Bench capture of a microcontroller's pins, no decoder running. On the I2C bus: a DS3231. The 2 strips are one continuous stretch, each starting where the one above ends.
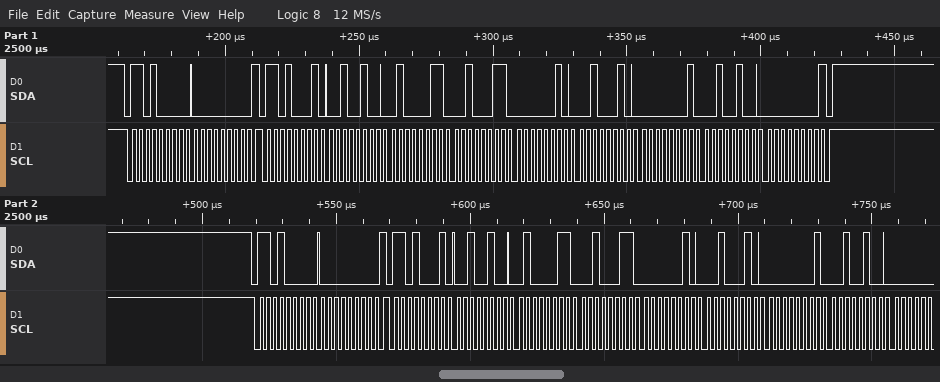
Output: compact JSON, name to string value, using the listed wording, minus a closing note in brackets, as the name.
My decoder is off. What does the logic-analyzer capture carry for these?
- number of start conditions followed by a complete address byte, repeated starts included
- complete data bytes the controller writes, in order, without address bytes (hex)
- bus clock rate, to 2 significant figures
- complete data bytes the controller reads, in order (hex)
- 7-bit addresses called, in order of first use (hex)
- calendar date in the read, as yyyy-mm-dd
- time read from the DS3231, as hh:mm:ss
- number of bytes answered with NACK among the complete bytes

{"number of start conditions followed by a complete address byte, repeated starts included": "4", "complete data bytes the controller writes, in order, without address bytes": "00 00", "bus clock rate, to 2 significant figures": "400 kHz", "complete data bytes the controller reads, in order": "24 43 23 02 22 01 24 00 24 43 23 02 22 01 24", "7-bit addresses called, in order of first use": "0x68", "calendar date in the read, as yyyy-mm-dd": "2024-01-22", "time read from the DS3231, as hh:mm:ss": "23:43:24", "number of bytes answered with NACK among the complete bytes": "1"}
